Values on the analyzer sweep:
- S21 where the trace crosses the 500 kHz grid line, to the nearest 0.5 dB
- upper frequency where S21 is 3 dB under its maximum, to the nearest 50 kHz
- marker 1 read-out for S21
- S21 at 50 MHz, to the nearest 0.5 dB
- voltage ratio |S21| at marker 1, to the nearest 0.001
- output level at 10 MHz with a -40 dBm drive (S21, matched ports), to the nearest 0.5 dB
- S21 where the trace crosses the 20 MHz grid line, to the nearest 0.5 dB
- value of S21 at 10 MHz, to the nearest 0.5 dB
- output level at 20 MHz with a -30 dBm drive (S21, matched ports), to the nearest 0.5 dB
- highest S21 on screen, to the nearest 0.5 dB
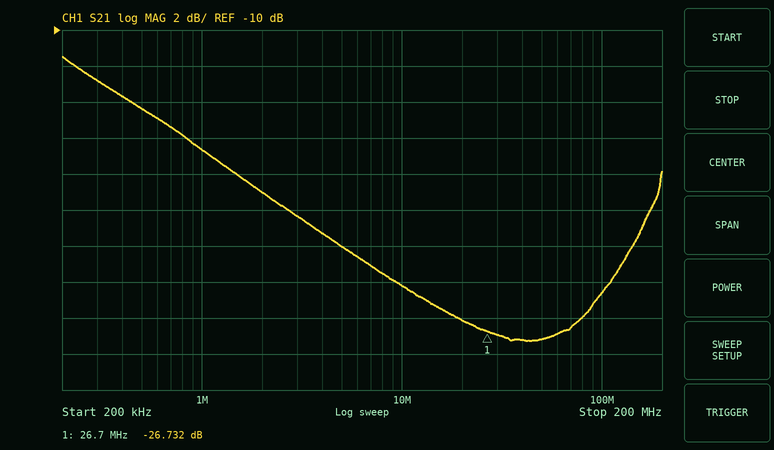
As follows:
-14.5 dB
500 kHz
-26.732 dB
-27.0 dB
0.046
-64.0 dBm
-26.0 dB
-24.0 dB
-56.0 dBm
-11.5 dB
